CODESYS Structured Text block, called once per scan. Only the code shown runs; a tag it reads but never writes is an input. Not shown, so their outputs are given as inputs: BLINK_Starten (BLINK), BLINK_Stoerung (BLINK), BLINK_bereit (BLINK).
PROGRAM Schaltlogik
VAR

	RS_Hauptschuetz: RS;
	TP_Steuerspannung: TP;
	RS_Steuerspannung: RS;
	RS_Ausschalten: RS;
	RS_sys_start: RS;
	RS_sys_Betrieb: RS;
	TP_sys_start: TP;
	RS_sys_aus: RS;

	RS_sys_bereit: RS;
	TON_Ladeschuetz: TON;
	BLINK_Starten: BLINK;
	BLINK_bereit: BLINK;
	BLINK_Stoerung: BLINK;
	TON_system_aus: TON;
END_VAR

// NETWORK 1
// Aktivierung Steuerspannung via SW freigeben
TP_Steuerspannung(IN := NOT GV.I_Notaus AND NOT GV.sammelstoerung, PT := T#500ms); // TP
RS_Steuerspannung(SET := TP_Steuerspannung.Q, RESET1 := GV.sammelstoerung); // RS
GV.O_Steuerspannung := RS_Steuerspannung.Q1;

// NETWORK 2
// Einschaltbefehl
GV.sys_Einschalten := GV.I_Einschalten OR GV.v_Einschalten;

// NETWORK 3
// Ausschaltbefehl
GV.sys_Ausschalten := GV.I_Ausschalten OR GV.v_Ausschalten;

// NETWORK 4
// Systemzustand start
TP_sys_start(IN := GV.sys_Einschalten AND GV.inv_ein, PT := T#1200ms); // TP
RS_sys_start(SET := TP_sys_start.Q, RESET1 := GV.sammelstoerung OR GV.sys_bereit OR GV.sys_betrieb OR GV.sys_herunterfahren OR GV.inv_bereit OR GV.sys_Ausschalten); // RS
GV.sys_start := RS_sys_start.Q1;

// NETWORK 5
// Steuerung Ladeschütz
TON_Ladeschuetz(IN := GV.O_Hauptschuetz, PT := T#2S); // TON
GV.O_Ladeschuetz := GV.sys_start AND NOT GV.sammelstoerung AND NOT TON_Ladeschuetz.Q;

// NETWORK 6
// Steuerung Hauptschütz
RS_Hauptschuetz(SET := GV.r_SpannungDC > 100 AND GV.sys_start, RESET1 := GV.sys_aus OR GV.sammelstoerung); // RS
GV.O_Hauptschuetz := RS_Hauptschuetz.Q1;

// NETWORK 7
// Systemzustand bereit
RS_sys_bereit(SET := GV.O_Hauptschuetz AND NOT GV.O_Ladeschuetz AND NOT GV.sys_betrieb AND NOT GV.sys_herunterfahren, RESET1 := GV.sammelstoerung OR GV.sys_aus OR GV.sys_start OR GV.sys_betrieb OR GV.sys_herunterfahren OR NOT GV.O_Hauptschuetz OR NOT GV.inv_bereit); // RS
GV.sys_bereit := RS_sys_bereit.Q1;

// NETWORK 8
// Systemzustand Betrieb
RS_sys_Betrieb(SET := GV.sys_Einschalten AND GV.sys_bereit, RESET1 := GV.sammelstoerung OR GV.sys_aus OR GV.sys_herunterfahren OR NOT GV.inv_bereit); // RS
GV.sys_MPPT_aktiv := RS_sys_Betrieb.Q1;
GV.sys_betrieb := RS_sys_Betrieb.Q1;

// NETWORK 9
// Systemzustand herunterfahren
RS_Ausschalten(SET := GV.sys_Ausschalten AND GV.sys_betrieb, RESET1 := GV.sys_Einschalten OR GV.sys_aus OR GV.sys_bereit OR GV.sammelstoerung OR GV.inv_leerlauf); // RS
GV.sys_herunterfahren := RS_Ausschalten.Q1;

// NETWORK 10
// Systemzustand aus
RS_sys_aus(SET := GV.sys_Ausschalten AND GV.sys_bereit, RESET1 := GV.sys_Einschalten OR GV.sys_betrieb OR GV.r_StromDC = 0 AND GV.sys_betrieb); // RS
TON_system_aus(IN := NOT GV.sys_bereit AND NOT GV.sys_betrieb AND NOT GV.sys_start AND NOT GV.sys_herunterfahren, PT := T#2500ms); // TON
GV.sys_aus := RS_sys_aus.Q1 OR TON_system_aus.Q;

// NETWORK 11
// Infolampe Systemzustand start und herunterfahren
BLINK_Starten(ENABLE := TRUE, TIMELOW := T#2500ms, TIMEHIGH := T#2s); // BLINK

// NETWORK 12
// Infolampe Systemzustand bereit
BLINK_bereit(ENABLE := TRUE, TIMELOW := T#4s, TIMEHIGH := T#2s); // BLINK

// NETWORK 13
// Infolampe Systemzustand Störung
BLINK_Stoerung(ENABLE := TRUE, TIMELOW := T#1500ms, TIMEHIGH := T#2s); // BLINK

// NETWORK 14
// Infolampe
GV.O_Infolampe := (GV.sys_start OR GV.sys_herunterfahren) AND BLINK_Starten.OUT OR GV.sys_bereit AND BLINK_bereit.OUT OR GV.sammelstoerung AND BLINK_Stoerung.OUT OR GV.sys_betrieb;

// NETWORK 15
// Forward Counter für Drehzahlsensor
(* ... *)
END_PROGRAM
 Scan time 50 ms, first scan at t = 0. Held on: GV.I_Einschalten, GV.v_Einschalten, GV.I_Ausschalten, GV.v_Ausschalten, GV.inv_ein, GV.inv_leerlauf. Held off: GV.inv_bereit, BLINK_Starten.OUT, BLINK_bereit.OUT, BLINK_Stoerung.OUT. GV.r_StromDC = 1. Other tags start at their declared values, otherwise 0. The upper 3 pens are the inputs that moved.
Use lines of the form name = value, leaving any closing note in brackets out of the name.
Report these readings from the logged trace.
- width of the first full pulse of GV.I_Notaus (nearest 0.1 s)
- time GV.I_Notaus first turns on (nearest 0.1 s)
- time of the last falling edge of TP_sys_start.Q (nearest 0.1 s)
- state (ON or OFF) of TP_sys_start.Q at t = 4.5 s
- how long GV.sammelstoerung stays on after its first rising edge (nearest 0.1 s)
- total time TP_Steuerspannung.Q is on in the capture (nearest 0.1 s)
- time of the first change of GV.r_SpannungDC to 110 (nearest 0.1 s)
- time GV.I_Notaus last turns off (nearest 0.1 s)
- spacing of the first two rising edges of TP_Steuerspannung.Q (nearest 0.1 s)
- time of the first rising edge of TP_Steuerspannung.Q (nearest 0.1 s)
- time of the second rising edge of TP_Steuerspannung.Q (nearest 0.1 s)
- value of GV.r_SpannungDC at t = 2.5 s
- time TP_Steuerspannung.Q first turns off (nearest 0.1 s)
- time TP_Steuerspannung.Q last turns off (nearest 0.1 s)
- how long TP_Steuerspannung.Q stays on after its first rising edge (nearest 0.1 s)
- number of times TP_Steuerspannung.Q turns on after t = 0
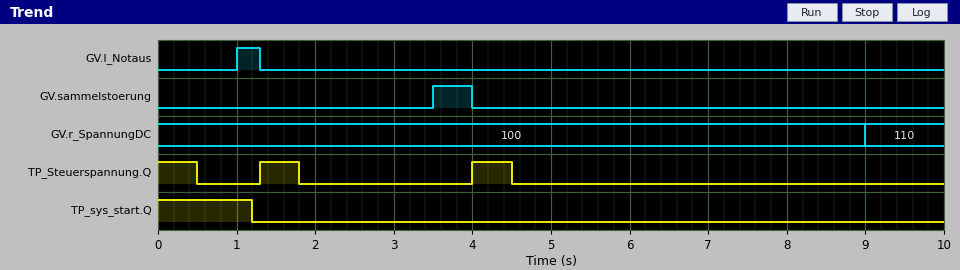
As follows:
width of the first full pulse of GV.I_Notaus = 0.3 s
time GV.I_Notaus first turns on = 1.0 s
time of the last falling edge of TP_sys_start.Q = 1.2 s
state (ON or OFF) of TP_sys_start.Q at t = 4.5 s = OFF
how long GV.sammelstoerung stays on after its first rising edge = 0.5 s
total time TP_Steuerspannung.Q is on in the capture = 1.5 s
time of the first change of GV.r_SpannungDC to 110 = 9.0 s
time GV.I_Notaus last turns off = 1.3 s
spacing of the first two rising edges of TP_Steuerspannung.Q = 2.7 s
time of the first rising edge of TP_Steuerspannung.Q = 1.3 s
time of the second rising edge of TP_Steuerspannung.Q = 4.0 s
value of GV.r_SpannungDC at t = 2.5 s = 100
time TP_Steuerspannung.Q first turns off = 0.5 s
time TP_Steuerspannung.Q last turns off = 4.5 s
how long TP_Steuerspannung.Q stays on after its first rising edge = 0.5 s
number of times TP_Steuerspannung.Q turns on after t = 0 = 2
